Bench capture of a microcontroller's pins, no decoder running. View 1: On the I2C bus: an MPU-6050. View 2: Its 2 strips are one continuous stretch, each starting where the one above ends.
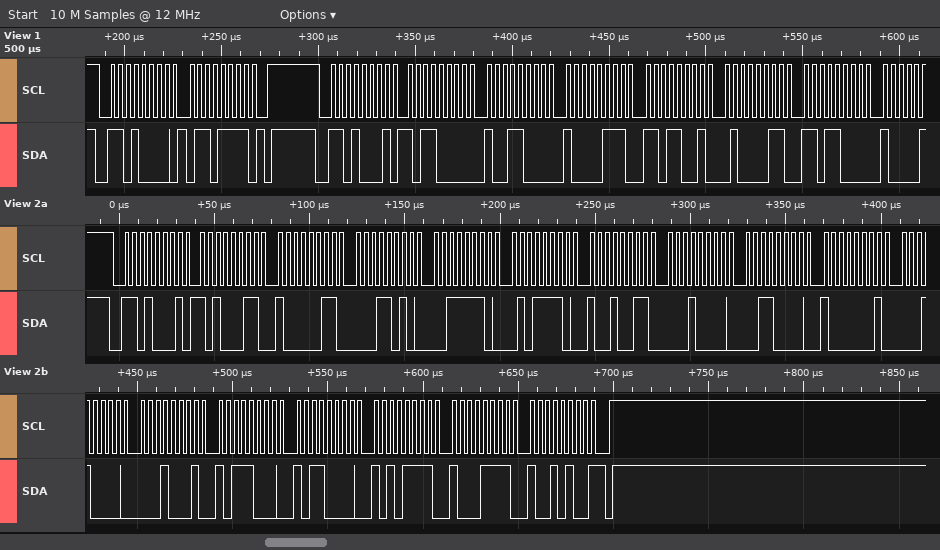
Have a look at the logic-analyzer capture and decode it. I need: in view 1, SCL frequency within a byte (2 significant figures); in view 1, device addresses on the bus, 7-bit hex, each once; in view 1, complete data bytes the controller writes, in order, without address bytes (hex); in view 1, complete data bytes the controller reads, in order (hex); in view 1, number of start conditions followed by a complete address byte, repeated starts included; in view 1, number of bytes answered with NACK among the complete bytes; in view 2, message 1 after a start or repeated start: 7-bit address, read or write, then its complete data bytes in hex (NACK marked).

250 kHz
0x68
6F
B0 98 87 D9 43 D8
2
0
0x68 read: A3 83 1A 3E 5E 93 10 30 81 10 11 B8 B0 AF 8F 94 NACK
